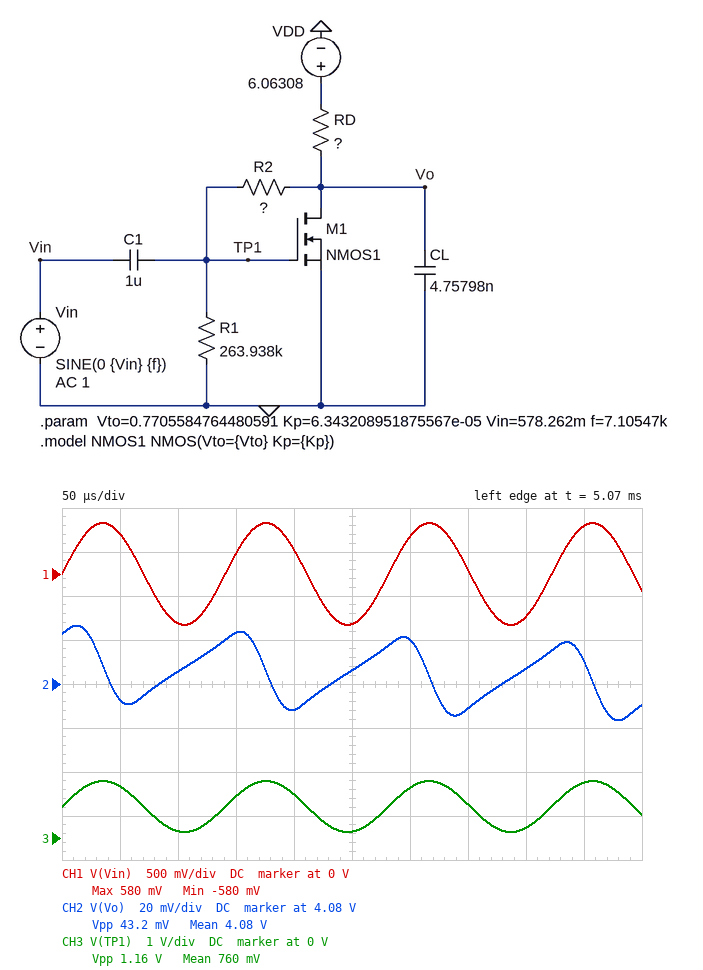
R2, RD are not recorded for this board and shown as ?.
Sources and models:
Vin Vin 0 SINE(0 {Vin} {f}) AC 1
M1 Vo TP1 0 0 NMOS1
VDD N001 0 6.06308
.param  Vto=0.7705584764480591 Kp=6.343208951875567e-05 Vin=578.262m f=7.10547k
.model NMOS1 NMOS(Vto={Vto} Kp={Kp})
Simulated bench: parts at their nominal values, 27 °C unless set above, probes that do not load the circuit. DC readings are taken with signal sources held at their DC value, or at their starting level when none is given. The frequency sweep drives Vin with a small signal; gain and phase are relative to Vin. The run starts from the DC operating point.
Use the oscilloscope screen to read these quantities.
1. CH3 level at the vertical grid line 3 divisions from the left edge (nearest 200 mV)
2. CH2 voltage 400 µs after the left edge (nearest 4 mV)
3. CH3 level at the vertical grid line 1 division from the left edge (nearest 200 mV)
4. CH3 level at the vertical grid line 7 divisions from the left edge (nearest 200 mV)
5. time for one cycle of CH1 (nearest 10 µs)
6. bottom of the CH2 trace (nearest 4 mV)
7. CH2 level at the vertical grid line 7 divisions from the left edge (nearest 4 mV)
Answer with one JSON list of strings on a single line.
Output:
["1.0 V", "4.088 V", "1.2 V", "800 mV", "140 µs", "4.064 V", "4.068 V"]
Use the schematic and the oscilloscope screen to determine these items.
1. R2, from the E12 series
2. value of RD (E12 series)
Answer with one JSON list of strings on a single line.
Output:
["1.5 MΩ", "470 kΩ"]
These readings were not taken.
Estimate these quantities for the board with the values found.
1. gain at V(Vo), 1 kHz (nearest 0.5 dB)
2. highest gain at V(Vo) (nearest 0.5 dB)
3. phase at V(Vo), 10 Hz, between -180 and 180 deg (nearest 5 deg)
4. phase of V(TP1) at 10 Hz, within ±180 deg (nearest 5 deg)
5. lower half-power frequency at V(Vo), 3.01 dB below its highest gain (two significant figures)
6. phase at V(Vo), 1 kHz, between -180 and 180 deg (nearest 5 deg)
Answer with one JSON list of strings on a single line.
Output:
["-33.0 dB", "-12.5 dB", "0 deg", "5 deg", "670 mHz", "-85 deg"]
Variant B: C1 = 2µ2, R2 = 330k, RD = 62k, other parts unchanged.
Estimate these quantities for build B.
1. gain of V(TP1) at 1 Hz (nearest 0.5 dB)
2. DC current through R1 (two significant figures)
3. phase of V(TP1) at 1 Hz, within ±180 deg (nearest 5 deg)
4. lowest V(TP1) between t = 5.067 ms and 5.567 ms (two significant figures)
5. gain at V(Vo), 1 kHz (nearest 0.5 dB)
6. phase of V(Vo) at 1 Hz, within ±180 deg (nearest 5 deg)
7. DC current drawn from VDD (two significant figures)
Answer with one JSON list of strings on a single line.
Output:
["-3.5 dB", "6.5 µA", "50 deg", "1.1 V", "4.0 dB", "-130 deg", "35 µA"]
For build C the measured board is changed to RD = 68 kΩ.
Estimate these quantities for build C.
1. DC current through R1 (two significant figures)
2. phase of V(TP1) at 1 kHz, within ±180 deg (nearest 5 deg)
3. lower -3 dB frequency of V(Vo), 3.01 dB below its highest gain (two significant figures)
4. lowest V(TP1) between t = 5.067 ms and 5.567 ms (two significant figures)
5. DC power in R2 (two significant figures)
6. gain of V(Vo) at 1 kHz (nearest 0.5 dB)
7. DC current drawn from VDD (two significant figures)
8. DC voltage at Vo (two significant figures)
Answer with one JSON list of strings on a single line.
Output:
["3.3 µA", "0 deg", "750 mHz", "290 mV", "16 µW", "-15.5 dB", "3.6 µA", "5.8 V"]
